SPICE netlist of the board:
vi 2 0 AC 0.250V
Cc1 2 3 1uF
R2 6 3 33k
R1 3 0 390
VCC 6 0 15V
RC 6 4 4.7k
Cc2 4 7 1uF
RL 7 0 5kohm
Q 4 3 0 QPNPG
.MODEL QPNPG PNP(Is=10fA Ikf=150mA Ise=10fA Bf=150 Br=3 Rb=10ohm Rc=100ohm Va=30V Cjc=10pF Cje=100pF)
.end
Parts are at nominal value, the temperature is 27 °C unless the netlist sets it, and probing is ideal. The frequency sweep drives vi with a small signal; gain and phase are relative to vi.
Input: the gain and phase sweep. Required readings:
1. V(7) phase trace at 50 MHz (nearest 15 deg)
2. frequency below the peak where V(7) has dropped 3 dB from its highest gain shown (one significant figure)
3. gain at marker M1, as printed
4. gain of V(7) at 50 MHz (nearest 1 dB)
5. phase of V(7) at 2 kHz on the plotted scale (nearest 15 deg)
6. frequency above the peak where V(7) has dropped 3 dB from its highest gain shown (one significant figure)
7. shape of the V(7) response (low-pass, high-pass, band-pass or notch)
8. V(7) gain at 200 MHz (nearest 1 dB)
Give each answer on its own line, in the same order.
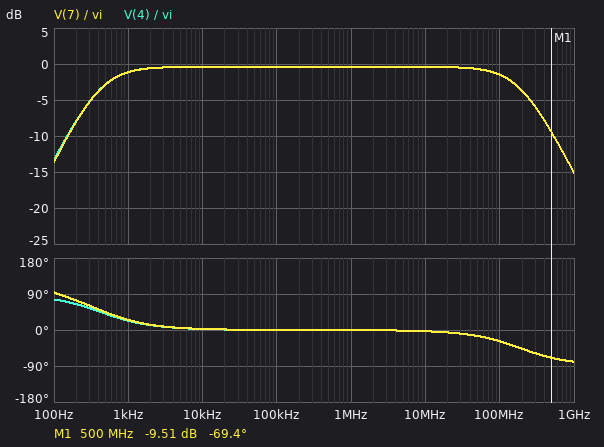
-15 deg
400 Hz
-9.51 dB
-1 dB
15 deg
200 MHz
band-pass
-4 dB
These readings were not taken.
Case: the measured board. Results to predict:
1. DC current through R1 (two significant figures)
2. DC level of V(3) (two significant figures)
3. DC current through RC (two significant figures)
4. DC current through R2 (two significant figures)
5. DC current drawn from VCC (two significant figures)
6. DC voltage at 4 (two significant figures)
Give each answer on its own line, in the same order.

1.2 mA
460 mV
2.9 mA
440 µA
3.3 mA
1.4 V
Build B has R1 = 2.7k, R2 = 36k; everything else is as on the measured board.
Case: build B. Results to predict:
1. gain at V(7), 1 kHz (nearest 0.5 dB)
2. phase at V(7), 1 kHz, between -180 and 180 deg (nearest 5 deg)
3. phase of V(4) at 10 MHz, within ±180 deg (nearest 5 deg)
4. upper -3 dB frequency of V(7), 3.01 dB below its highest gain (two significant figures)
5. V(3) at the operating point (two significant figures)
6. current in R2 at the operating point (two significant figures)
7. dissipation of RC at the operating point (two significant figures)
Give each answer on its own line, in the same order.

-0.5 dB
5 deg
0 deg
260 MHz
2.6 V
340 µA
28 mW
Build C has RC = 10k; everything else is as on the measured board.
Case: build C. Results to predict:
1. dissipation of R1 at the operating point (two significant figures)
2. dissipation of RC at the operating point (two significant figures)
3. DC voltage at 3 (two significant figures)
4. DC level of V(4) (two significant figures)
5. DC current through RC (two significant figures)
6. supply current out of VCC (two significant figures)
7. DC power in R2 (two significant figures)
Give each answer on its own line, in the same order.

250 µW
19 mW
310 mV
1.1 V
1.4 mA
1.8 mA
6.5 mW
